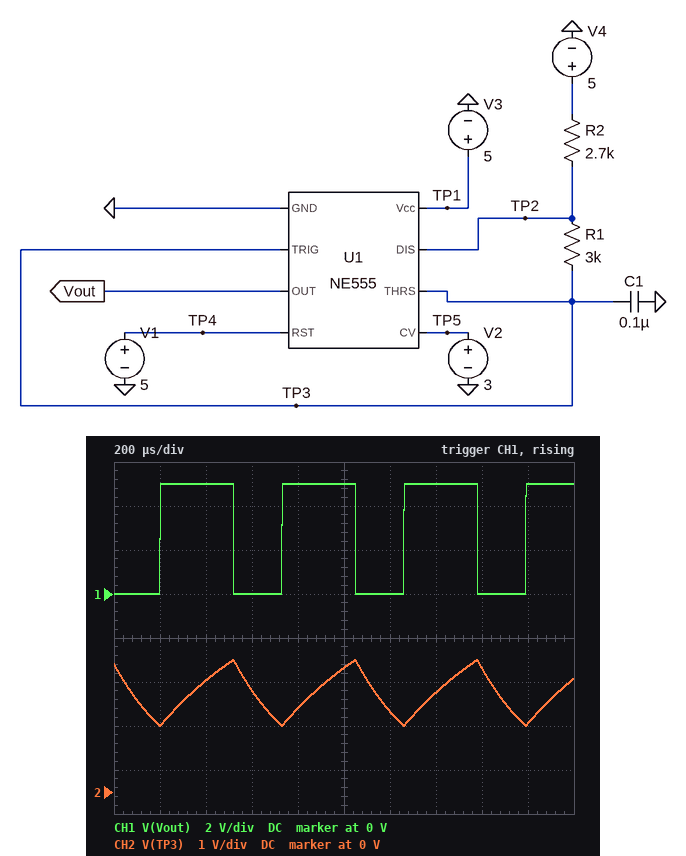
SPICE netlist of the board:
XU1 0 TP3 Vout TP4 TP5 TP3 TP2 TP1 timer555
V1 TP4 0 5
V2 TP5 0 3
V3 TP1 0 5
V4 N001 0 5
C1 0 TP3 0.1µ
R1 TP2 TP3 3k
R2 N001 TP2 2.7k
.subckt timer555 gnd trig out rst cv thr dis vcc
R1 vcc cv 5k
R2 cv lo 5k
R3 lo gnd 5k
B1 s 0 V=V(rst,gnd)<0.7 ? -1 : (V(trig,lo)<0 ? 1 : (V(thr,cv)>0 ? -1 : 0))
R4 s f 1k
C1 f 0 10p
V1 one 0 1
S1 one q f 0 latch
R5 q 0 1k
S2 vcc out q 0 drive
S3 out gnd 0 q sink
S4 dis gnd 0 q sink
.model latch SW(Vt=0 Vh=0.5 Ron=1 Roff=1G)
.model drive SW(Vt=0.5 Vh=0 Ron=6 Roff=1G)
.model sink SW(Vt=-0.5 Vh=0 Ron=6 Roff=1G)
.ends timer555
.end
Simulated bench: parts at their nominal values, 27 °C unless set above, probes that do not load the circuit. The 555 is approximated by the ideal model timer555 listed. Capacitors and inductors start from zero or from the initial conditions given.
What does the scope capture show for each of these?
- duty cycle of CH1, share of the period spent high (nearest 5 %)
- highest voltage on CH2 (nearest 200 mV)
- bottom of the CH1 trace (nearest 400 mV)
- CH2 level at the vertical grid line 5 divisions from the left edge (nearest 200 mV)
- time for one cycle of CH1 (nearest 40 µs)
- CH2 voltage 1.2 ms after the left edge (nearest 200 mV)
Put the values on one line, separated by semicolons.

60 %; 3.0 V; 0 V; 2.8 V; 520 µs; 1.8 V
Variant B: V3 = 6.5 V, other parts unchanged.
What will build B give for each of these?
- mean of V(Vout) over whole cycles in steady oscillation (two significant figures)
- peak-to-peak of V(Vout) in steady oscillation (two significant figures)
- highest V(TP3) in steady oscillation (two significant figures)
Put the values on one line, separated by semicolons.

3.9 V; 6.5 V; 3.0 V
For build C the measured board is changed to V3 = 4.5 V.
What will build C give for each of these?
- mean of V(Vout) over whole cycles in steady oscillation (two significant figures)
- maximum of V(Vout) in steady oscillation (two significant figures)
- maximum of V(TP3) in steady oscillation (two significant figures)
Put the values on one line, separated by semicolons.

2.7 V; 4.5 V; 3.0 V
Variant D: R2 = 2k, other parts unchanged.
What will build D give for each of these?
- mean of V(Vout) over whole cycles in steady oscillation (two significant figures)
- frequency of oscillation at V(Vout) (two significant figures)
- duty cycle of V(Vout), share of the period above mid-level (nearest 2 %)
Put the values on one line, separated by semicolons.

2.9 V; 2.0 kHz; 58 %
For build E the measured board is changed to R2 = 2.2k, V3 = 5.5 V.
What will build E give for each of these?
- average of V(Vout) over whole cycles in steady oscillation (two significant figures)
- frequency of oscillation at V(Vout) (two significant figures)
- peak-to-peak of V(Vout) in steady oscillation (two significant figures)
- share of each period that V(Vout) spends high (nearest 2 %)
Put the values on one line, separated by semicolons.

3.2 V; 2.0 kHz; 5.5 V; 58 %
